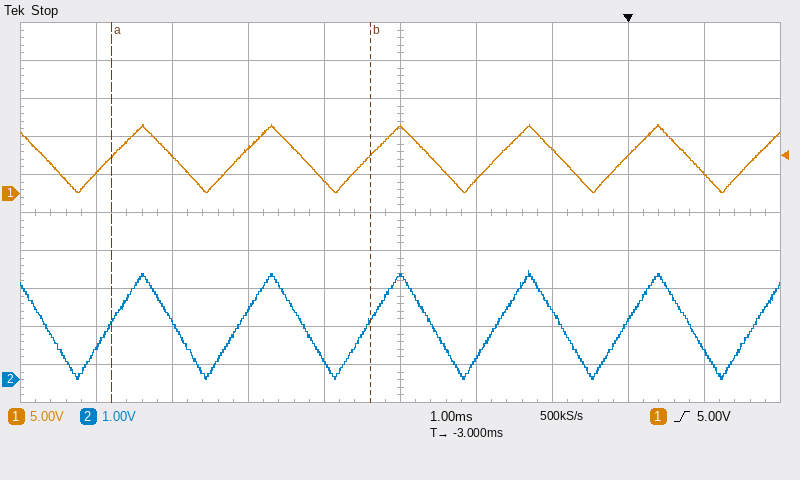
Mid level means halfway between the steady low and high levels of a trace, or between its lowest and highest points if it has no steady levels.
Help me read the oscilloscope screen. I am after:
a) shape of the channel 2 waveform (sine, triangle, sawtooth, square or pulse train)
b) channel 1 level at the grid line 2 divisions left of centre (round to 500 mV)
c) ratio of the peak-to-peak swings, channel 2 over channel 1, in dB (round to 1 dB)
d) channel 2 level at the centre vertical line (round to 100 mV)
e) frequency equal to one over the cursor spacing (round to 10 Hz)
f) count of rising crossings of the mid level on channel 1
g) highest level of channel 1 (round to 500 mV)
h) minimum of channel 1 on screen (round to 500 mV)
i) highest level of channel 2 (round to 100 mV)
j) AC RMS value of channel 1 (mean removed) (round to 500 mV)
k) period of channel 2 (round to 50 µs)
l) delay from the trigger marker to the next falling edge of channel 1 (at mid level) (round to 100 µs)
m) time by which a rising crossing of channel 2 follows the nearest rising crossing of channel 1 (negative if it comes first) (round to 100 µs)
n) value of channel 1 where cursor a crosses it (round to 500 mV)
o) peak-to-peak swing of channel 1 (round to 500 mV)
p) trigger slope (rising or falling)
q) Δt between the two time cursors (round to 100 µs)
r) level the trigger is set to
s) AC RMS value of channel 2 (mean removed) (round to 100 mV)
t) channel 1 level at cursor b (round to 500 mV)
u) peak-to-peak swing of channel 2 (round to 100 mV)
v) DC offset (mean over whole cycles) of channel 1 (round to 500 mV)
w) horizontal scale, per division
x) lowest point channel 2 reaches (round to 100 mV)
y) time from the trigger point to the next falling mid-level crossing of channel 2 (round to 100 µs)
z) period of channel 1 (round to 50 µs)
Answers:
triangle
6.0 V
-10 dB
2.7 V
290 Hz
6
9.0 V
0.0 V
2.9 V
2.5 V
1.70 ms
800 µs
0.0 ms
5.0 V
9.0 V
rising
3.4 ms
5.00 V
800 mV
5.0 V
2.9 V
4.5 V
1 ms
0.0 V
800 µs
1.70 ms
